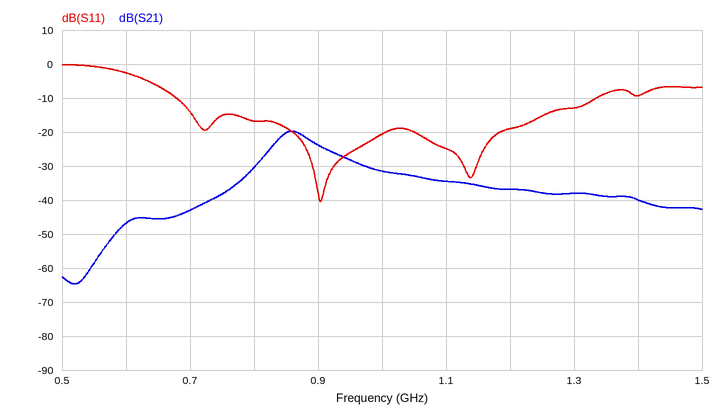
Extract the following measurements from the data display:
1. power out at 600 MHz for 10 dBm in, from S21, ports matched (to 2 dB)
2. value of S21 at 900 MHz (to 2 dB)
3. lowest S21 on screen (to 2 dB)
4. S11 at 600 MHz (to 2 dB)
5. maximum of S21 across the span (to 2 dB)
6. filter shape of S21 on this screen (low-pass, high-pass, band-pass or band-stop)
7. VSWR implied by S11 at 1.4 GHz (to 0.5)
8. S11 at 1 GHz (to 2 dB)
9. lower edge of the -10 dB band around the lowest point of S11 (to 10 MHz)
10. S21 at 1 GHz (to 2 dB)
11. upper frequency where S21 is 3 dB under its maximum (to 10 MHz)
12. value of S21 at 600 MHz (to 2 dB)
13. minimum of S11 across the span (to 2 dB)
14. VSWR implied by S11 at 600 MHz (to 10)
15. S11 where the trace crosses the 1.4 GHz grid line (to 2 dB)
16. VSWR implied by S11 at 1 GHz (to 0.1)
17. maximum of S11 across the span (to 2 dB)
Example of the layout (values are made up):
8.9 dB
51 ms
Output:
-36 dBm
-24 dB
-64 dB
-2 dB
-20 dB
band-pass
2.0
-20 dB
680 MHz
-32 dB
890 MHz
-46 dB
-40 dB
10
-10 dB
1.2
0 dB
